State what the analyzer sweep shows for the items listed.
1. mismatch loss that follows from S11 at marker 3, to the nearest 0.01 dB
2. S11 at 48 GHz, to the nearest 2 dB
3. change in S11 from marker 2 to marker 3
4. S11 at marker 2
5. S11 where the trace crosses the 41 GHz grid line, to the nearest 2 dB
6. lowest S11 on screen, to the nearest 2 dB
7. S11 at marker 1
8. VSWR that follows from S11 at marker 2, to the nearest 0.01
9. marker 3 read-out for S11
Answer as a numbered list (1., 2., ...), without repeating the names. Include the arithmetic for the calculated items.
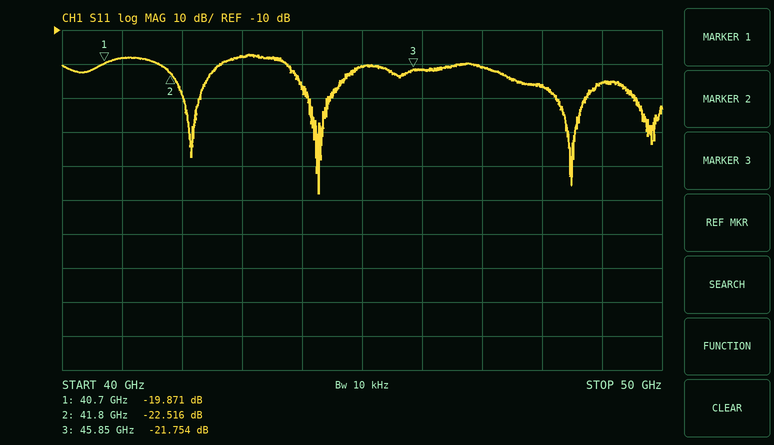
1. −10 log10(1 − 10^(-21.754/10)) ≈ 0.03 dB
2. -26 dB
3. -21.754 − (-22.516) = 0.762 dB
4. -22.516 dB
5. -18 dB
6. -58 dB
7. -19.871 dB
8. (1 + 0.0749)/(1 − 0.0749) ≈ 1.16
9. -21.754 dB
